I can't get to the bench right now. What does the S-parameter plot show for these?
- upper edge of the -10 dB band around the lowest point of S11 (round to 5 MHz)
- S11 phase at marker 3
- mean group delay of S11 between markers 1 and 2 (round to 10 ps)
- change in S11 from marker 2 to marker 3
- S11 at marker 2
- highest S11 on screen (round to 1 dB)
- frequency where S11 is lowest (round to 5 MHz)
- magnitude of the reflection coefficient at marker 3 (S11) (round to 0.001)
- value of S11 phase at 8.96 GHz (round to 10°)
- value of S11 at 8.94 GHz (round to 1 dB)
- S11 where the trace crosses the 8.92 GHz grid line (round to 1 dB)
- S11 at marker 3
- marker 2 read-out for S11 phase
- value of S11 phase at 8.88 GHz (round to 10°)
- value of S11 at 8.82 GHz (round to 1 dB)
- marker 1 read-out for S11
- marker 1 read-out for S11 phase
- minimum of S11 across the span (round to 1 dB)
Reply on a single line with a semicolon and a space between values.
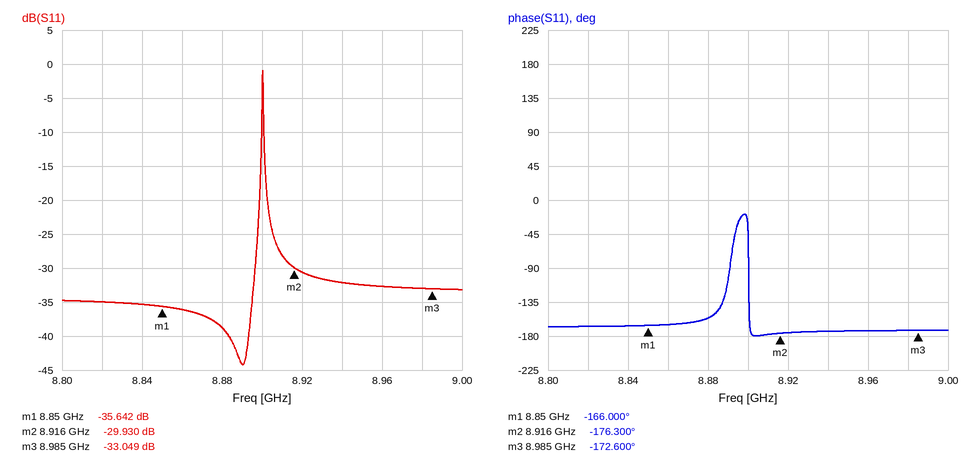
8.900 GHz; -172.600°; 430 ps; -3.119 dB; -29.930 dB; -1 dB; 8.890 GHz; 0.022; -170°; -32 dB; -31 dB; -33.049 dB; -176.300°; -160°; -35 dB; -35.642 dB; -166.000°; -44 dB
